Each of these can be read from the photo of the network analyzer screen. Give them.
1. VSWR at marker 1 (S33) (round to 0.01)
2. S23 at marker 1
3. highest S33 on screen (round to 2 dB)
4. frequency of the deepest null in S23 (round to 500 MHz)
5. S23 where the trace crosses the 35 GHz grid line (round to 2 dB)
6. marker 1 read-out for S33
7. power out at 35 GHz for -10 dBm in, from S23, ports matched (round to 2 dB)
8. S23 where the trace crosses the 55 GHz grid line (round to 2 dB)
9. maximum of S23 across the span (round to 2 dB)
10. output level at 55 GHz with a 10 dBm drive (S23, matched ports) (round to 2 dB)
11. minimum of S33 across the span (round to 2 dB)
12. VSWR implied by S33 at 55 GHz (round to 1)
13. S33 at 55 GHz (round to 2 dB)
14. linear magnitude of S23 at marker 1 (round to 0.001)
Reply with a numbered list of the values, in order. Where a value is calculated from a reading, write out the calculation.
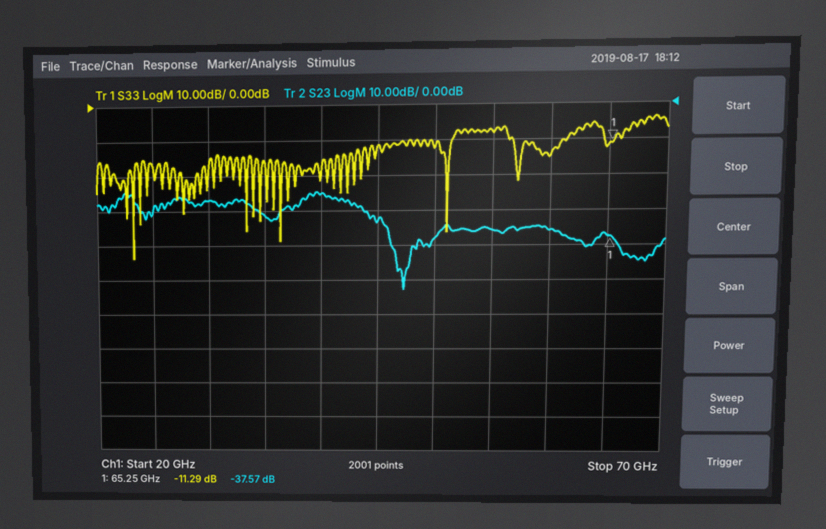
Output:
1. (1 + 0.2726)/(1 − 0.2726) ≈ 1.75
2. -37.57 dB
3. -4 dB
4. 47.5 GHz
5. -32 dB
6. -11.29 dB
7. -10 dBm + (-32 dB) = -42 dBm
8. -36 dB
9. -24 dB
10. 10 dBm + (-36 dB) = -26 dBm
11. -44 dB
12. |Γ| = 10^(-8/20) = 0.3981; VSWR = (1 + 0.3981)/(1 − 0.3981) ≈ 2
13. -8 dB
14. 10^(-37.57/20) ≈ 0.013
